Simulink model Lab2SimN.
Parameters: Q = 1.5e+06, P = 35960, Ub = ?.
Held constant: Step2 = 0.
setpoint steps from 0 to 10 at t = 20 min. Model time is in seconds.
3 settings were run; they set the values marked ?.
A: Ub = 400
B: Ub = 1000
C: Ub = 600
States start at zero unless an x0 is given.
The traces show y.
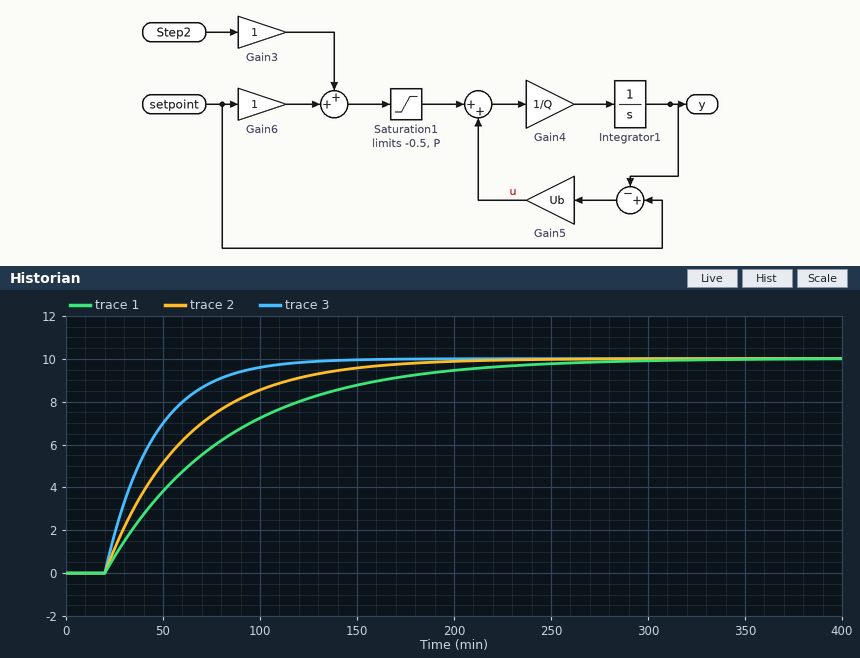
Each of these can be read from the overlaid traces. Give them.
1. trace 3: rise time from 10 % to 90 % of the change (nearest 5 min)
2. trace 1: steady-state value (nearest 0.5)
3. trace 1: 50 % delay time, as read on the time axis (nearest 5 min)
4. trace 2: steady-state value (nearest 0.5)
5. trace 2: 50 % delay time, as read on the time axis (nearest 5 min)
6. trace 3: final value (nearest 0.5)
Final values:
55 min
10.0
65 min
10.0
50 min
10.0
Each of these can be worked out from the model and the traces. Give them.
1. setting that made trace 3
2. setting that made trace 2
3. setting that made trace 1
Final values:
B
C
A
